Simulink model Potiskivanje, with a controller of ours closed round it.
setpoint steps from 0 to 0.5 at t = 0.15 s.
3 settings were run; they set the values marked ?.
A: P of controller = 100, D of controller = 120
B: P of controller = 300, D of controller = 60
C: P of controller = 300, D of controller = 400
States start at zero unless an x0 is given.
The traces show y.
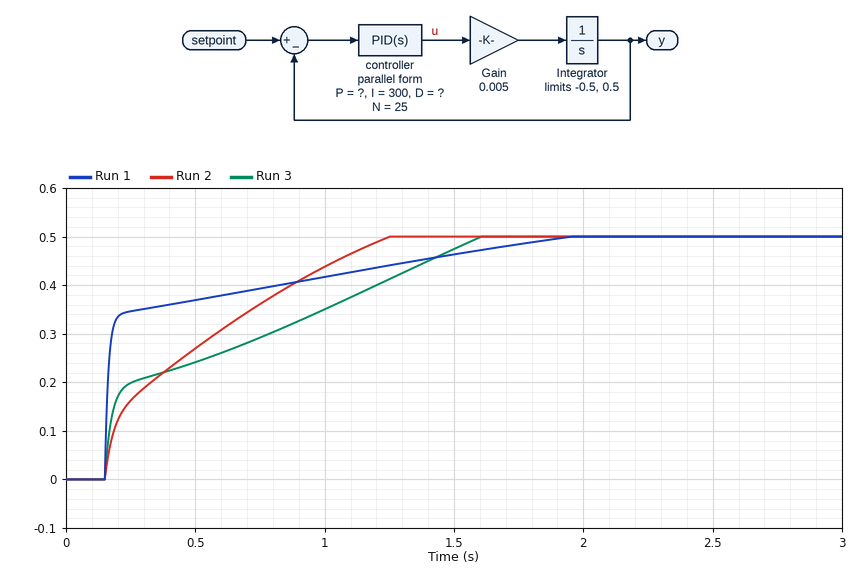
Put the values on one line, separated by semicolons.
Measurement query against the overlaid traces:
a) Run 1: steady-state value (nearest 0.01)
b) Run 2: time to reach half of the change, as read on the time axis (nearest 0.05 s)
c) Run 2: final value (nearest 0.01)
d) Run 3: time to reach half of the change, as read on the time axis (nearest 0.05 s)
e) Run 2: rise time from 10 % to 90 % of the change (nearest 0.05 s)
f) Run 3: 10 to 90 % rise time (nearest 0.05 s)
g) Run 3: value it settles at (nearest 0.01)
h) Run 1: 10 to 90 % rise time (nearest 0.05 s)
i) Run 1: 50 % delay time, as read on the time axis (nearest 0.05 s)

0.50; 0.45 s; 0.50; 0.55 s; 0.90 s; 1.25 s; 0.50; 1.20 s; 0.15 s
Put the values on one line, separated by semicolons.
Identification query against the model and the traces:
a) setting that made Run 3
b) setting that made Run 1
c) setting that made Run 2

A; C; B
